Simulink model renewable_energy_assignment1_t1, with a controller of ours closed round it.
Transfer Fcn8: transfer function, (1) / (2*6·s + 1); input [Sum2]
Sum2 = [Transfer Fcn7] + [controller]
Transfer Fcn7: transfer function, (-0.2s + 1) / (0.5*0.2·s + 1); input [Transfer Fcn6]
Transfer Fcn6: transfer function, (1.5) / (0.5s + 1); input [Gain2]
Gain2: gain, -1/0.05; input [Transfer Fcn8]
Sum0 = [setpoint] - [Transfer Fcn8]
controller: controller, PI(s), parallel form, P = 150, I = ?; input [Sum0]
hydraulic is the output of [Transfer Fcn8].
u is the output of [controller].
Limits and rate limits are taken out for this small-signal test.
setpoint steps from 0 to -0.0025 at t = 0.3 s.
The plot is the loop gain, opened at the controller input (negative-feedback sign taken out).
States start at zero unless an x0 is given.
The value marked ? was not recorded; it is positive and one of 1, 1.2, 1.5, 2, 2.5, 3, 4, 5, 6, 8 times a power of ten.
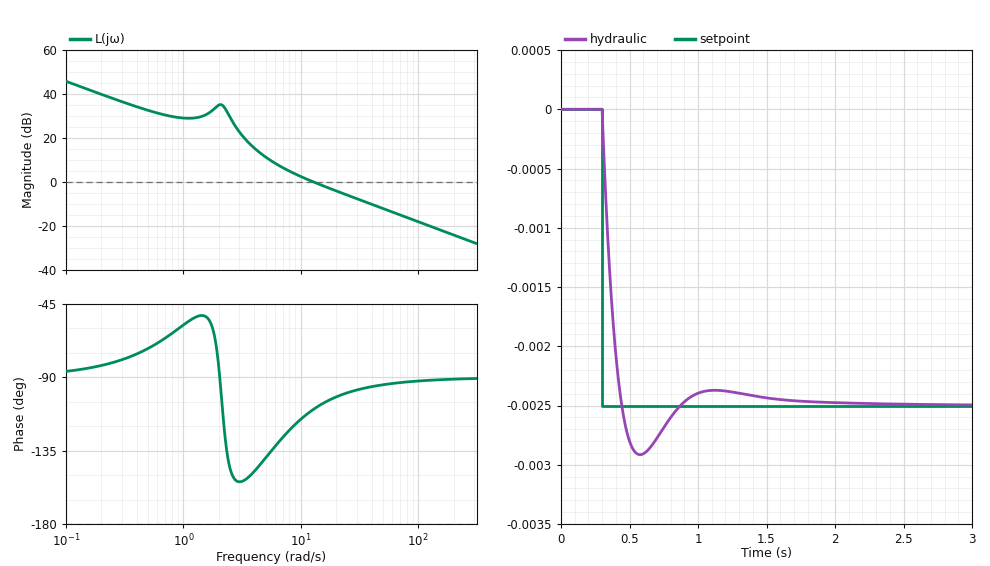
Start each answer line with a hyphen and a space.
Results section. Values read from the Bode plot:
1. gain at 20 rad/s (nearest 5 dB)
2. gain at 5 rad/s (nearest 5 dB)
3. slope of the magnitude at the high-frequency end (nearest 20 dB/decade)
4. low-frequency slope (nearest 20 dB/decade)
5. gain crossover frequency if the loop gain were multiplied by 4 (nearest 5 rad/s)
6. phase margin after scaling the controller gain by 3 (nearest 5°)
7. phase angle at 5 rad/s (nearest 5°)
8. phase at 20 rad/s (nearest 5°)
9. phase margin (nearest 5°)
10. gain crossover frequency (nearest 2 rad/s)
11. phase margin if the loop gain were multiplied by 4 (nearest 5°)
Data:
- -5 dB
- 10 dB
- -20 dB/decade
- -20 dB/decade
- 50 rad/s
- 85°
- -140°
- -100°
- 70°
- 12 rad/s
- 85°
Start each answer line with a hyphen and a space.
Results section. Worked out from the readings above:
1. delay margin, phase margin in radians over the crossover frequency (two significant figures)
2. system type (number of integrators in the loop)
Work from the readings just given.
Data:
- 0.10 s
- 1
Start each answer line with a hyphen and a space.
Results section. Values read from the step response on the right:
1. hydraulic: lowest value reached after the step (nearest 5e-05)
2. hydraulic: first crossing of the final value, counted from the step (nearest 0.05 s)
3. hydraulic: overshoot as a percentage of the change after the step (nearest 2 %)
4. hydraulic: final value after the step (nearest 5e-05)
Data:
- -0.00290
- 0.15 s
- 16 %
- -0.00250
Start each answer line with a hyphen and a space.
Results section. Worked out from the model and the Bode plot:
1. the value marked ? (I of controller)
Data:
- 600
